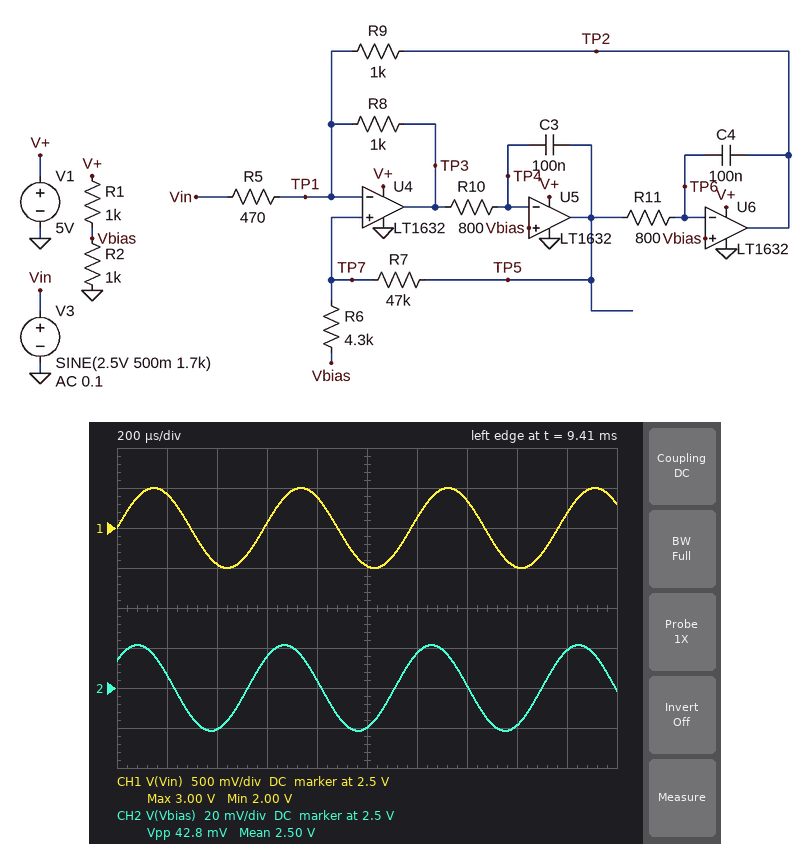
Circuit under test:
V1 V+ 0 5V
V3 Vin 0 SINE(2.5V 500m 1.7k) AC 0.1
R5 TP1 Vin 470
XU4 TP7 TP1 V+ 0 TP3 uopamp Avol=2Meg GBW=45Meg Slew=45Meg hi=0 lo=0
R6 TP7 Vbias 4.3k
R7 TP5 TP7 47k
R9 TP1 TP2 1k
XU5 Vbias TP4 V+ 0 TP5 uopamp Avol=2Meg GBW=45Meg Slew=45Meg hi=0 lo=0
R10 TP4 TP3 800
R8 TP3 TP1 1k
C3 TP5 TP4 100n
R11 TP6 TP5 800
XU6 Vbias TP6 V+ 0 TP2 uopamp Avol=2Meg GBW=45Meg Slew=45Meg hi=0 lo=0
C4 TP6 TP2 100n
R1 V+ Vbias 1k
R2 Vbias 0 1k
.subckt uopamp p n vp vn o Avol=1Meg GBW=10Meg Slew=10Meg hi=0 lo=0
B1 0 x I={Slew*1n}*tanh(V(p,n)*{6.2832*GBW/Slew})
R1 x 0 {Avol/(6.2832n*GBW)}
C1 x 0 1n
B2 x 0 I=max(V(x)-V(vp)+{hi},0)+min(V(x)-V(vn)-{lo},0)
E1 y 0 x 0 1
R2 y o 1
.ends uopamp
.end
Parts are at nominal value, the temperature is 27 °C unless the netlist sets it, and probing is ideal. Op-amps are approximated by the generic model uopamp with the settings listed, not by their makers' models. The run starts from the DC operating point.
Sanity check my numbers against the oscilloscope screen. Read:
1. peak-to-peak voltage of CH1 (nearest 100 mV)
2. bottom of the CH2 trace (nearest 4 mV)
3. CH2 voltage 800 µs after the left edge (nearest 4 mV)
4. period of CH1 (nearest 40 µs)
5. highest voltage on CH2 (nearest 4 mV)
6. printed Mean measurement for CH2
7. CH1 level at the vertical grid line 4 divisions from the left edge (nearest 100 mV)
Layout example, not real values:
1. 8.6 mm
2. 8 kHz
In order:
1. 1.0 V
2. 2.480 V
3. 2.504 V
4. 600 µs
5. 2.520 V
6. 2.50 V
7. 2.9 V
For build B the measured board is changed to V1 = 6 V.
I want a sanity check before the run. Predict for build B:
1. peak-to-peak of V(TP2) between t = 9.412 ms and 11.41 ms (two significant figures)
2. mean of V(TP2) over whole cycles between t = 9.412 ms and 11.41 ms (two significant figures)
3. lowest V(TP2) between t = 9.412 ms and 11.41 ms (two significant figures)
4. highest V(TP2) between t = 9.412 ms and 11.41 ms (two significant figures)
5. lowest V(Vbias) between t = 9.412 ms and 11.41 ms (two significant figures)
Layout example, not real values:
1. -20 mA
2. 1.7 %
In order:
1. 4.5 V
2. 4.0 V
3. 1.5 V
4. 6.0 V
5. 3.0 V
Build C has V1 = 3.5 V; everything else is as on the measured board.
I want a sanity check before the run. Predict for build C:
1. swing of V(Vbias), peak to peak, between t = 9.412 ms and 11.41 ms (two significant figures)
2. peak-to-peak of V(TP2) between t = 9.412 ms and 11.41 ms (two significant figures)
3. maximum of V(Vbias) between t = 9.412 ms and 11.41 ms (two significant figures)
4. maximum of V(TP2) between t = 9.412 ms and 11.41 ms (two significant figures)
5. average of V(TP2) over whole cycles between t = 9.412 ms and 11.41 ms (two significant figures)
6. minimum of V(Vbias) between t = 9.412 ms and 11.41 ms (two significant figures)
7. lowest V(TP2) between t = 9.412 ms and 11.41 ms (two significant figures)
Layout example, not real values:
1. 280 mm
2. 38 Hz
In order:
1. 28 mV
2. 1.5 V
3. 1.8 V
4. 1.4 V
5. 350 mV
6. 1.7 V
7. -44 mV
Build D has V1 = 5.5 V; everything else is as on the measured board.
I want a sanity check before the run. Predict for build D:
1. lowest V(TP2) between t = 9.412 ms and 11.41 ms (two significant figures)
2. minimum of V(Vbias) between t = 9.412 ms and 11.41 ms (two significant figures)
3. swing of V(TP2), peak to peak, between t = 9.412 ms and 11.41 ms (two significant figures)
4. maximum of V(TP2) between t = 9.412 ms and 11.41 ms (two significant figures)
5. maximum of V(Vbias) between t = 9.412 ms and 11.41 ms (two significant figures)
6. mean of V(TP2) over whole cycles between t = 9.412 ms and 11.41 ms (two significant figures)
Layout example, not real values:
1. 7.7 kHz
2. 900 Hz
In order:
1. 730 mV
2. 2.7 V
3. 4.8 V
4. 5.5 V
5. 2.8 V
6. 3.3 V
